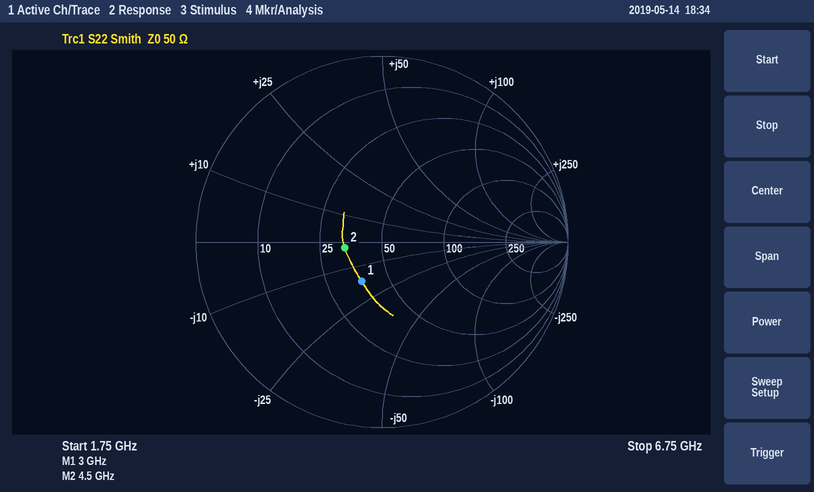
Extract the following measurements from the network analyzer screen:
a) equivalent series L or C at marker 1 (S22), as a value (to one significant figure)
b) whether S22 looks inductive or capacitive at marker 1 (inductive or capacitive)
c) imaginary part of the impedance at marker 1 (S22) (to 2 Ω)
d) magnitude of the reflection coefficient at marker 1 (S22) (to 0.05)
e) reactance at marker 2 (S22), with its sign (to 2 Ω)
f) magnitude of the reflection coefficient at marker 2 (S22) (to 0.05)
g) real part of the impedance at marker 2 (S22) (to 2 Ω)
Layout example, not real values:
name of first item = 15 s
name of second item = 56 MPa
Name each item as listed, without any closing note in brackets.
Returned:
equivalent series L or C at marker 1 (S22), as a value = 3 pF
whether S22 looks inductive or capacitive at marker 1 = capacitive
imaginary part of the impedance at marker 1 (S22) = -16 Ω
magnitude of the reflection coefficient at marker 1 (S22) = 0.25
reactance at marker 2 (S22), with its sign = -2 Ω
magnitude of the reflection coefficient at marker 2 (S22) = 0.20
real part of the impedance at marker 2 (S22) = 34 Ω
